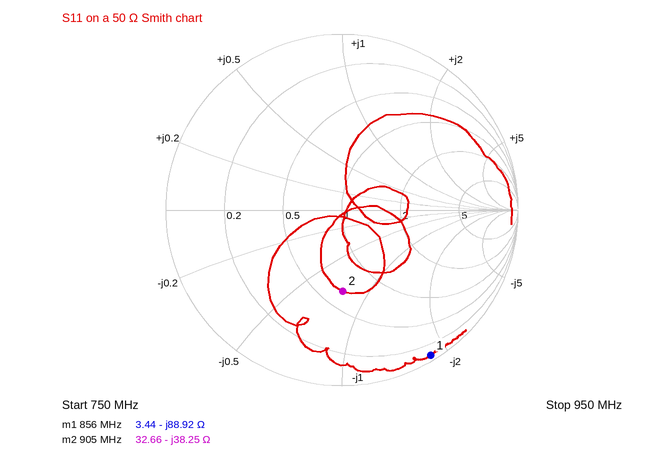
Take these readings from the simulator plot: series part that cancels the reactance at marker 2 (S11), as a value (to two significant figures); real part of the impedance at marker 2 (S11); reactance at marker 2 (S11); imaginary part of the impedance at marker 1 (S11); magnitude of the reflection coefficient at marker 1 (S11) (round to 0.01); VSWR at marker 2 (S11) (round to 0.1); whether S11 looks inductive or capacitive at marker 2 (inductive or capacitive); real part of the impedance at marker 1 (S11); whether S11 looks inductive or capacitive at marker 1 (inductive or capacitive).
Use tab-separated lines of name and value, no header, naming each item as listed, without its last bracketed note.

series part that cancels the reactance at marker 2 (S11), as a value	6.7 nH
real part of the impedance at marker 2	32.66 Ω
reactance at marker 2	-38.25 Ω
imaginary part of the impedance at marker 1	-88.92 Ω
magnitude of the reflection coefficient at marker 1 (S11)	0.97
VSWR at marker 2 (S11)	2.7
whether S11 looks inductive or capacitive at marker 2	capacitive
real part of the impedance at marker 1	3.44 Ω
whether S11 looks inductive or capacitive at marker 1	capacitive
